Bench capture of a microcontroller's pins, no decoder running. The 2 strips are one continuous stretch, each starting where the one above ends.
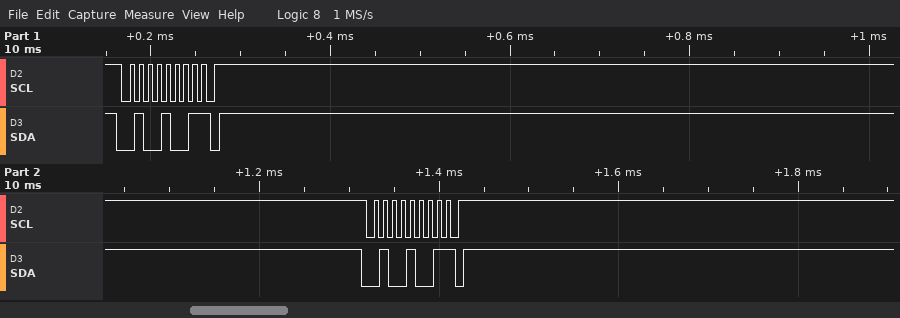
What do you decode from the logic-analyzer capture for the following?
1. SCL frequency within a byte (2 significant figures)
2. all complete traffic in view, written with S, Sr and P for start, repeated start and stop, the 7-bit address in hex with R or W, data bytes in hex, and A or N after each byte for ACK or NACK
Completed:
100 kHz
S 24R N P S 24R N P
